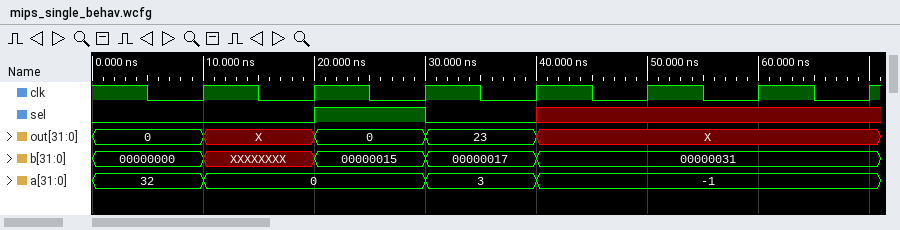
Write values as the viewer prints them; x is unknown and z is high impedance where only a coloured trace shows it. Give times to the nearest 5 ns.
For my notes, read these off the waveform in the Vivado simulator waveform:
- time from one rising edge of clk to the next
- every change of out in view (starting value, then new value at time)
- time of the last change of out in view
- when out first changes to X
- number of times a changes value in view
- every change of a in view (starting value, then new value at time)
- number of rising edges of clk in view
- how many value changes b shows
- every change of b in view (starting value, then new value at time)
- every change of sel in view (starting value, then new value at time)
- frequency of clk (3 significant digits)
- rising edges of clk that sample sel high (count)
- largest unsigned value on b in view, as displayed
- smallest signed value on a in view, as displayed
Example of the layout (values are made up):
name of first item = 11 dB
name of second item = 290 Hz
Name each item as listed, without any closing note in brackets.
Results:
time from one rising edge of clk to the next = 10 ns
every change of out in view = 0, X at 10 ns, 0 at 20 ns, 23 at 30 ns, X at 40 ns
time of the last change of out in view = 40 ns
when out first changes to X = 10 ns
number of times a changes value in view = 3
every change of a in view = 32, 0 at 10 ns, 3 at 30 ns, -1 at 40 ns
number of rising edges of clk in view = 7
how many value changes b shows = 4
every change of b in view = 00000000, XXXXXXXX at 10 ns, 00000015 at 20 ns, 00000017 at 30 ns, 00000031 at 40 ns
every change of sel in view = 0, 1 at 20 ns, 0 at 30 ns, x at 40 ns
frequency of clk = 100 MHz
rising edges of clk that sample sel high = 1
largest unsigned value on b in view, as displayed = 00000031
smallest signed value on a in view, as displayed = -1
